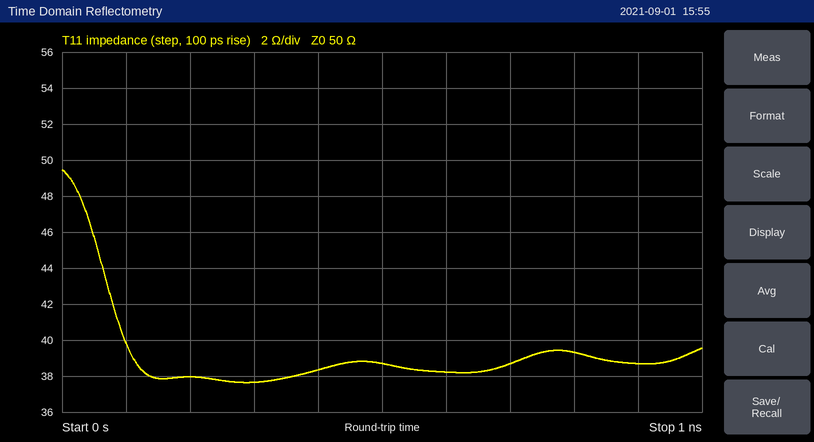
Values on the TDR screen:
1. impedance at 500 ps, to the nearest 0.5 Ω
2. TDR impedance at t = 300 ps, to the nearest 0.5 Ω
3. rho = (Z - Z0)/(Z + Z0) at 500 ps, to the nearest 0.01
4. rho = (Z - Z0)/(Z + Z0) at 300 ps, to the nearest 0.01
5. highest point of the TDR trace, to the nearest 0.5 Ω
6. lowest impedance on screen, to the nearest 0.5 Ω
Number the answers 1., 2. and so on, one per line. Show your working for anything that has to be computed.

1. 38.5 Ω
2. 37.5 Ω
3. (38.5 − 50)/(38.5 + 50) ≈ -0.13
4. (37.5 − 50)/(37.5 + 50) ≈ -0.14
5. 49.5 Ω
6. 37.5 Ω
